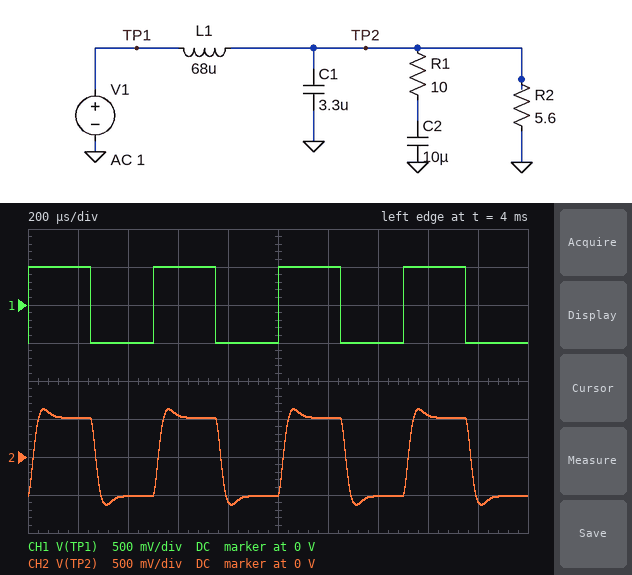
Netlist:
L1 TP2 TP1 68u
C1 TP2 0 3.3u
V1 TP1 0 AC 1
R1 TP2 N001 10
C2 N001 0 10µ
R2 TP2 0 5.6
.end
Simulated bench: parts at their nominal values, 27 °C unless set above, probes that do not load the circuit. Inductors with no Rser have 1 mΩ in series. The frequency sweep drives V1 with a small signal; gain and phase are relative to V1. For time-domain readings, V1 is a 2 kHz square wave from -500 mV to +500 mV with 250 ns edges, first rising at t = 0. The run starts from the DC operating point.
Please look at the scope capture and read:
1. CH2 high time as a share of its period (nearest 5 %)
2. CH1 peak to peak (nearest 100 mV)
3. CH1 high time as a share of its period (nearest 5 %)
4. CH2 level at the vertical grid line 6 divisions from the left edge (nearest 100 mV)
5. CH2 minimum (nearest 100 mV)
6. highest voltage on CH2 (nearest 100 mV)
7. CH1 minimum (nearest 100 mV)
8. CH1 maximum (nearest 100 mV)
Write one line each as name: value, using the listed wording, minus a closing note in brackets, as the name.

CH2 high time as a share of its period: 50 %
CH1 peak to peak: 1.0 V
CH1 high time as a share of its period: 50 %
CH2 level at the vertical grid line 6 divisions from the left edge: 500 mV
CH2 minimum: -600 mV
highest voltage on CH2: 600 mV
CH1 minimum: -500 mV
CH1 maximum: 500 mV
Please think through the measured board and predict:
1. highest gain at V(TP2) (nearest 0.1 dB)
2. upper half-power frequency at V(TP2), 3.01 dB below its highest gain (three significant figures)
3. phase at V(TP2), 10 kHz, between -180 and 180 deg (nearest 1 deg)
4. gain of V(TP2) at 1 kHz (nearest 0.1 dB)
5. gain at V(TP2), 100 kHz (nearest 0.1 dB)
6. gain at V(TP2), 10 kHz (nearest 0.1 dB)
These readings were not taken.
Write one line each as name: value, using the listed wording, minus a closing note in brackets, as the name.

highest gain at V(TP2): 0.7 dB
upper half-power frequency at V(TP2), 3.01 dB below its highest gain: 10.9 kHz
phase at V(TP2), 10 kHz, between -180 and 180 deg: -88 deg
gain of V(TP2) at 1 kHz: 0.2 dB
gain at V(TP2), 100 kHz: -38.9 dB
gain at V(TP2), 10 kHz: -1.4 dB
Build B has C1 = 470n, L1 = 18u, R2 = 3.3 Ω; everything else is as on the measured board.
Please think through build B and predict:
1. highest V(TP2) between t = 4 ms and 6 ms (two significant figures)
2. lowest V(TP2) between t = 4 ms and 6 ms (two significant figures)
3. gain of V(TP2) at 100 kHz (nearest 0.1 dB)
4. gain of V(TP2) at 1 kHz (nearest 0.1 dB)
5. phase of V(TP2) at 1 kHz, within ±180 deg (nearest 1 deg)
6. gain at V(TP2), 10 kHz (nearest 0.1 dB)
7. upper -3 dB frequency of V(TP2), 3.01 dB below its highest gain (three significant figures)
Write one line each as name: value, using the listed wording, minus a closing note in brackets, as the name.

highest V(TP2) between t = 4 ms and 6 ms: 510 mV
lowest V(TP2) between t = 4 ms and 6 ms: -510 mV
gain of V(TP2) at 100 kHz: -14.2 dB
gain of V(TP2) at 1 kHz: 0 dB
phase of V(TP2) at 1 kHz, within ±180 deg: -2 deg
gain at V(TP2), 10 kHz: -0.4 dB
upper -3 dB frequency of V(TP2), 3.01 dB below its highest gain: 25.9 kHz
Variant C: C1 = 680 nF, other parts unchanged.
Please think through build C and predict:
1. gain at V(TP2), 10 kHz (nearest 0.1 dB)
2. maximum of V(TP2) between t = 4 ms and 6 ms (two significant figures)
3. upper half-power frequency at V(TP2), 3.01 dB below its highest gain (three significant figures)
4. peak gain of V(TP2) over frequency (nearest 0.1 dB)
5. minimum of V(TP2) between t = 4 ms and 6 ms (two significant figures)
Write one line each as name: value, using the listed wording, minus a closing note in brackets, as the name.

gain at V(TP2), 10 kHz: -2.9 dB
maximum of V(TP2) between t = 4 ms and 6 ms: 530 mV
upper half-power frequency at V(TP2), 3.01 dB below its highest gain: 9.72 kHz
peak gain of V(TP2) over frequency: 0.2 dB
minimum of V(TP2) between t = 4 ms and 6 ms: -530 mV
